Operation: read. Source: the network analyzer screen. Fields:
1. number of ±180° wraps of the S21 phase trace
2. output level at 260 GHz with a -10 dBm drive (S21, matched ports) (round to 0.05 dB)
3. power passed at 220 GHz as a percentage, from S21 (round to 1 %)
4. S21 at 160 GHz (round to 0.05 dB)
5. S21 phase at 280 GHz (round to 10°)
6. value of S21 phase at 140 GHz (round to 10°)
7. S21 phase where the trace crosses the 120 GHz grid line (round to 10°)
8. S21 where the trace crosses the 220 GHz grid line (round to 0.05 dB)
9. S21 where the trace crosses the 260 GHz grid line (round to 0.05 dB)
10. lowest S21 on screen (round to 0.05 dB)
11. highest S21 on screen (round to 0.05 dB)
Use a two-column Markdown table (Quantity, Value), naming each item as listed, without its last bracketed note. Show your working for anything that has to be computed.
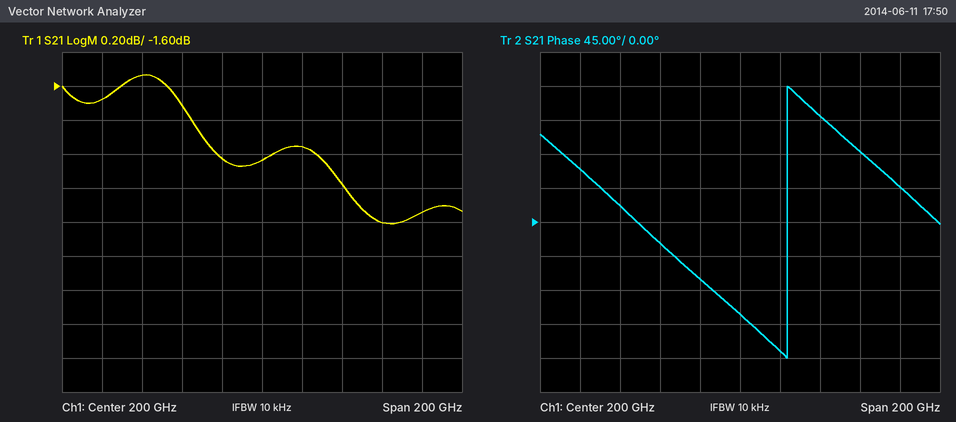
| Quantity | Value |
|---|---|
| number of ±180° wraps of the S21 phase trace | 1 |
| output level at 260 GHz with a -10 dBm drive (S21, matched ports) | -10 dBm + (-2.40 dB) = -12.40 dBm |
| power passed at 220 GHz as a percentage, from S21 | 10^(-1.95/10) ≈ 64 % |
| S21 at 160 GHz | -1.70 dB |
| S21 phase at 280 GHz | 50° |
| value of S21 phase at 140 GHz | 20° |
| S21 phase where the trace crosses the 120 GHz grid line | 70° |
| S21 where the trace crosses the 220 GHz grid line | -1.95 dB |
| S21 where the trace crosses the 260 GHz grid line | -2.40 dB |
| lowest S21 on screen | -2.40 dB |
| highest S21 on screen | -1.55 dB |
